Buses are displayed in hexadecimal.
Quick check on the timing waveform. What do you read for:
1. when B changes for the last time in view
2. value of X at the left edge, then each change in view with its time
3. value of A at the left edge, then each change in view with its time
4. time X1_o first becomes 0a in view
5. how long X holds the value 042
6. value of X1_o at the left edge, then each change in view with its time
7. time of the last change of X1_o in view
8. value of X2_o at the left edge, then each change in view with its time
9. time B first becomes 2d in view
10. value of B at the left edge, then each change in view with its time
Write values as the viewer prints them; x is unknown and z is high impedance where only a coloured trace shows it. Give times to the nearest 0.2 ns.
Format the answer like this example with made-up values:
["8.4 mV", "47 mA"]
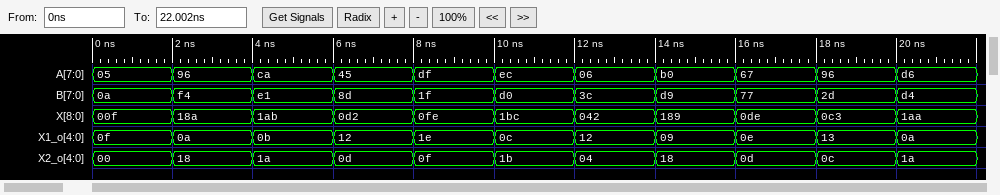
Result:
["20 ns", "00f, 18a at 2 ns, 1ab at 4 ns, 0d2 at 6 ns, 0fe at 8 ns, 1bc at 10 ns, 042 at 12 ns, 189 at 14 ns, 0de at 16 ns, 0c3 at 18 ns, 1aa at 20 ns", "05, 96 at 2 ns, ca at 4 ns, 45 at 6 ns, df at 8 ns, ec at 10 ns, 06 at 12 ns, b0 at 14 ns, 67 at 16 ns, 96 at 18 ns, d6 at 20 ns", "2 ns", "2 ns", "0f, 0a at 2 ns, 0b at 4 ns, 12 at 6 ns, 1e at 8 ns, 0c at 10 ns, 12 at 12 ns, 09 at 14 ns, 0e at 16 ns, 13 at 18 ns, 0a at 20 ns", "20 ns", "00, 18 at 2 ns, 1a at 4 ns, 0d at 6 ns, 0f at 8 ns, 1b at 10 ns, 04 at 12 ns, 18 at 14 ns, 0d at 16 ns, 0c at 18 ns, 1a at 20 ns", "18 ns", "0a, f4 at 2 ns, e1 at 4 ns, 8d at 6 ns, 1f at 8 ns, d0 at 10 ns, 3c at 12 ns, d9 at 14 ns, 77 at 16 ns, 2d at 18 ns, d4 at 20 ns"]
